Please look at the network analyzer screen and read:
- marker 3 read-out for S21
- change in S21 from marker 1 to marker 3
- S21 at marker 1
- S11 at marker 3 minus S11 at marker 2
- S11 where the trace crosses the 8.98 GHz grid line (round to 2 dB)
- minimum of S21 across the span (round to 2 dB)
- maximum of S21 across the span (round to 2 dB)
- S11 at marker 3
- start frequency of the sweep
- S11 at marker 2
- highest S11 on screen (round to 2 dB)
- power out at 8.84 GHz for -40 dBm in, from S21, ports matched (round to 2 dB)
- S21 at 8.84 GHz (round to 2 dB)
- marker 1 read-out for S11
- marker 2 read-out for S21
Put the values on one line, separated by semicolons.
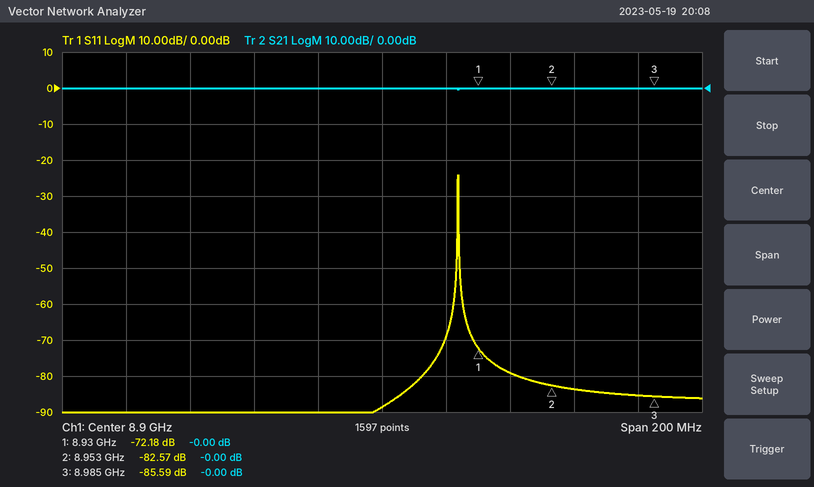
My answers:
-0.00 dB; 0.00 dB; -0.00 dB; -3.02 dB; -86 dB; 0 dB; 0 dB; -85.59 dB; 8.8 GHz; -82.57 dB; -24 dB; -40 dBm; 0 dB; -72.18 dB; -0.00 dB
